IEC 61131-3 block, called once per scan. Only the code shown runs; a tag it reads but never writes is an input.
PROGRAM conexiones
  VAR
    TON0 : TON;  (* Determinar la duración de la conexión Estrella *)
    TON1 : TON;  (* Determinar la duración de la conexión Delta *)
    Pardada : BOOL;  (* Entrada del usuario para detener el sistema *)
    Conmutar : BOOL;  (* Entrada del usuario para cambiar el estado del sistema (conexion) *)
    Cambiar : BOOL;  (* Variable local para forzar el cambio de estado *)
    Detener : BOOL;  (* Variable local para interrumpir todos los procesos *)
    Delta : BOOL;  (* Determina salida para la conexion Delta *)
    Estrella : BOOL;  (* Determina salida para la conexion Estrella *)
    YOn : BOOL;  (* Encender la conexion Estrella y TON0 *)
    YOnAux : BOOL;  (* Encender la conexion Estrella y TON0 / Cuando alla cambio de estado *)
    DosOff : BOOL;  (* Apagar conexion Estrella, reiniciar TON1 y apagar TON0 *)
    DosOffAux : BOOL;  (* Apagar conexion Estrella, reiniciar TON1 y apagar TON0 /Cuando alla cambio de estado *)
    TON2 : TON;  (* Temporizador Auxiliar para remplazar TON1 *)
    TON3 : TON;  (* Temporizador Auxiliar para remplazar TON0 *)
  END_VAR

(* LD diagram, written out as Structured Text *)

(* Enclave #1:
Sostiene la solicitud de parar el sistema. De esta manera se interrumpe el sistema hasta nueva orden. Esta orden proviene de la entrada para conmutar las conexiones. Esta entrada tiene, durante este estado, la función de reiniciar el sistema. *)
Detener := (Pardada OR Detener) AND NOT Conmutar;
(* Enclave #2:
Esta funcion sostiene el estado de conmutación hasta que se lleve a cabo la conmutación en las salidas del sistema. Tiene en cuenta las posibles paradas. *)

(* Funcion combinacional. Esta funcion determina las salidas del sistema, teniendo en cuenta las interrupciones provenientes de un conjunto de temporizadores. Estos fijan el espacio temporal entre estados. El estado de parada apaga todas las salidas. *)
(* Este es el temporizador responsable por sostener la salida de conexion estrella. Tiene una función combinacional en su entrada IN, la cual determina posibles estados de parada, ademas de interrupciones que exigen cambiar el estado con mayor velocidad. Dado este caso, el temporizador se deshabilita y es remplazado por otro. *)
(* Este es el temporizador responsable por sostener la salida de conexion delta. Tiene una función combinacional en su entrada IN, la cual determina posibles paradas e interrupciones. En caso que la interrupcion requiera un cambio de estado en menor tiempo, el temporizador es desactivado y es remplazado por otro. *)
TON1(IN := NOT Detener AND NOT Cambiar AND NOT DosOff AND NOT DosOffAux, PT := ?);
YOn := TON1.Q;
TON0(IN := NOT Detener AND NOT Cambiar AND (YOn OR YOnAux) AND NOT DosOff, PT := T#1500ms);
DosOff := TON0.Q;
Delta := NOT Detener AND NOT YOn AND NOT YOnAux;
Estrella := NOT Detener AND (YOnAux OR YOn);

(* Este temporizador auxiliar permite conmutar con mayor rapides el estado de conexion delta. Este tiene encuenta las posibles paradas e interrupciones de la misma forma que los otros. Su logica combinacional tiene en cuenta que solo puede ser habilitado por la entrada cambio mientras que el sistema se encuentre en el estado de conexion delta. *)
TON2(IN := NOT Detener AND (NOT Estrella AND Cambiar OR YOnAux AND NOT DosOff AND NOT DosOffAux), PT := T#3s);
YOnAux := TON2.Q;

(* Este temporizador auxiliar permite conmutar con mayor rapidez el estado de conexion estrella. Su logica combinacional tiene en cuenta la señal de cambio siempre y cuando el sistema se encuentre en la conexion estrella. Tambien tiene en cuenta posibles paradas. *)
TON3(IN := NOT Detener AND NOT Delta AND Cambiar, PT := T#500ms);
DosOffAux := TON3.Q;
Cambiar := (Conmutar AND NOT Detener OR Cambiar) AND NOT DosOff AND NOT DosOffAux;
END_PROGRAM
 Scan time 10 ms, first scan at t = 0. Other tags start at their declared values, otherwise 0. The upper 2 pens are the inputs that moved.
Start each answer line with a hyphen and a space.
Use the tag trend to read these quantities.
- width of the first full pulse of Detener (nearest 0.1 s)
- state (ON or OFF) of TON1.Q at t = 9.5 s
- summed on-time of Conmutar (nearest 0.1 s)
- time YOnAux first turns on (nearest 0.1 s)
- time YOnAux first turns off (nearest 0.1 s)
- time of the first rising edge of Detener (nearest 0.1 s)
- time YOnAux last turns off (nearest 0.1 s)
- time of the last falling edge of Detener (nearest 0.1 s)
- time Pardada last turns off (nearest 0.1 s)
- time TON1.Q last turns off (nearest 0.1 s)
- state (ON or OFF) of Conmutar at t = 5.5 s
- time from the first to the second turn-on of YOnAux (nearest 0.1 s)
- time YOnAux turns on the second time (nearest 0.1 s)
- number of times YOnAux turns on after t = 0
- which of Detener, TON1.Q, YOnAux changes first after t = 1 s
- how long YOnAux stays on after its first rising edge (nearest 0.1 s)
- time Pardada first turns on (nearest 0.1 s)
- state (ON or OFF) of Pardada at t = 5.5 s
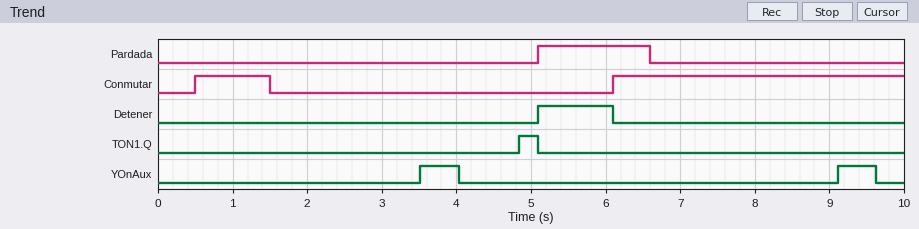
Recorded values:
- 1.0 s
- OFF
- 4.9 s
- 3.5 s
- 4.0 s
- 5.1 s
- 9.6 s
- 6.1 s
- 6.6 s
- 5.1 s
- OFF
- 5.6 s
- 9.1 s
- 2
- YOnAux
- 0.5 s
- 5.1 s
- ON
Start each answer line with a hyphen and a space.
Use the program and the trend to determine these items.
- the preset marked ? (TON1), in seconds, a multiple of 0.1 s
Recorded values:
- 0.8 s
